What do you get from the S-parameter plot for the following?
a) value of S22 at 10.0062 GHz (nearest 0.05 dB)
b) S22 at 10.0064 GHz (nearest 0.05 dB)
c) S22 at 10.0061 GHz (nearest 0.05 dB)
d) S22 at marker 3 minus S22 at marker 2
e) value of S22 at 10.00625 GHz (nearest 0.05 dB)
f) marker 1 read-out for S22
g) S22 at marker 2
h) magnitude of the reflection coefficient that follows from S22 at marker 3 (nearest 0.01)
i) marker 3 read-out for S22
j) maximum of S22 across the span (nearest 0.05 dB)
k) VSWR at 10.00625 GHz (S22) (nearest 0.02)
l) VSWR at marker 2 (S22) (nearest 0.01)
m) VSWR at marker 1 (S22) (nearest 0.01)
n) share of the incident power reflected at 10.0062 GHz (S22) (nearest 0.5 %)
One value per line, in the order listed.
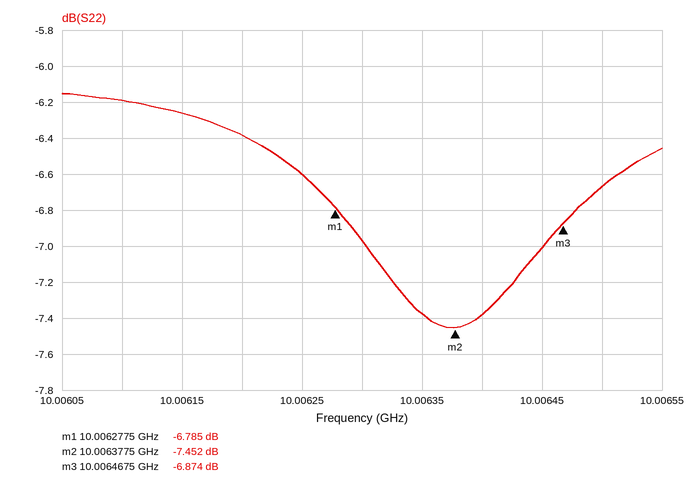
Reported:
-6.40 dB
-7.40 dB
-6.20 dB
0.578 dB
-6.60 dB
-6.785 dB
-7.452 dB
0.45
-6.874 dB
-6.15 dB
2.76
2.47
2.69
23.0 %
